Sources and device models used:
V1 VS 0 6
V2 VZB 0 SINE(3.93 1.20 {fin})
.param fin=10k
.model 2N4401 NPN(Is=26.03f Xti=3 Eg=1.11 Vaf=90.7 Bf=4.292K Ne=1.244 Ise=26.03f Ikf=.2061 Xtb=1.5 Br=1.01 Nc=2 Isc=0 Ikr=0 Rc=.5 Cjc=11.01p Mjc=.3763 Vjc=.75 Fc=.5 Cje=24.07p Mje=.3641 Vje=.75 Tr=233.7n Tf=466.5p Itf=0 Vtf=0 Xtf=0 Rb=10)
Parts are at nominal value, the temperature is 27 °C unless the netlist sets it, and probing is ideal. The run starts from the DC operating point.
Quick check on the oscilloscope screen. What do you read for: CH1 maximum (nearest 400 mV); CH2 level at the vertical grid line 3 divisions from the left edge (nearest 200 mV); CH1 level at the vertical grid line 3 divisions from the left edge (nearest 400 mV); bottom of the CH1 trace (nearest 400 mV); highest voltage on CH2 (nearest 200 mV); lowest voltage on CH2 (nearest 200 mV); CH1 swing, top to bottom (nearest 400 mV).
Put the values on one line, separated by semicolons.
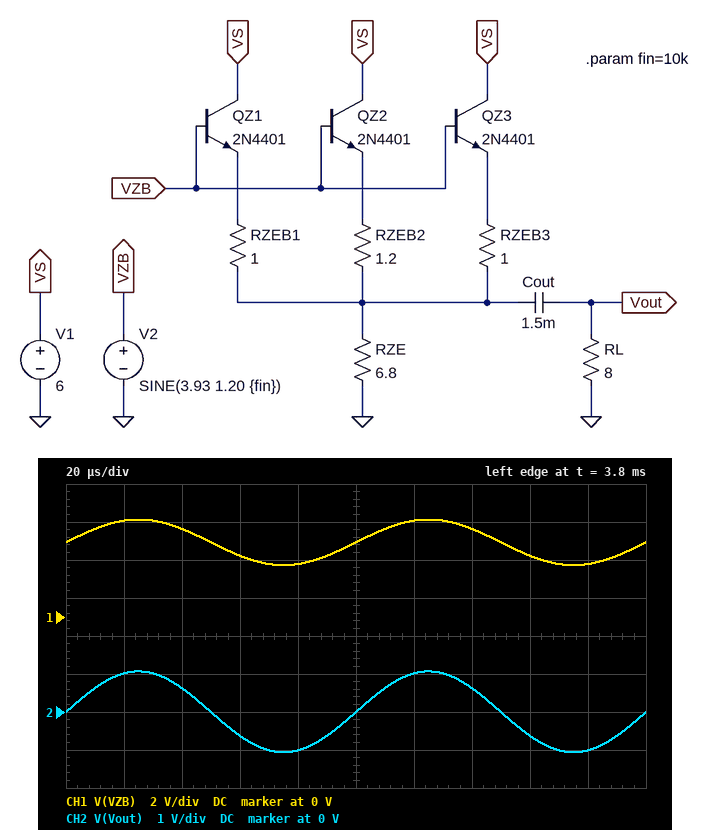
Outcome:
5.2 V; -600 mV; 3.2 V; 2.8 V; 1.0 V; -1.0 V; 2.4 V
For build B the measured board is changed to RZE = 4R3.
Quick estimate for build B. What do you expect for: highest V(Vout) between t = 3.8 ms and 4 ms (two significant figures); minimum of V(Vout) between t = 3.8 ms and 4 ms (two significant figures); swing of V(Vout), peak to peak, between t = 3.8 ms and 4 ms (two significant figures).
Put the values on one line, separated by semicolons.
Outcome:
1.0 V; -1.0 V; 2.1 V
